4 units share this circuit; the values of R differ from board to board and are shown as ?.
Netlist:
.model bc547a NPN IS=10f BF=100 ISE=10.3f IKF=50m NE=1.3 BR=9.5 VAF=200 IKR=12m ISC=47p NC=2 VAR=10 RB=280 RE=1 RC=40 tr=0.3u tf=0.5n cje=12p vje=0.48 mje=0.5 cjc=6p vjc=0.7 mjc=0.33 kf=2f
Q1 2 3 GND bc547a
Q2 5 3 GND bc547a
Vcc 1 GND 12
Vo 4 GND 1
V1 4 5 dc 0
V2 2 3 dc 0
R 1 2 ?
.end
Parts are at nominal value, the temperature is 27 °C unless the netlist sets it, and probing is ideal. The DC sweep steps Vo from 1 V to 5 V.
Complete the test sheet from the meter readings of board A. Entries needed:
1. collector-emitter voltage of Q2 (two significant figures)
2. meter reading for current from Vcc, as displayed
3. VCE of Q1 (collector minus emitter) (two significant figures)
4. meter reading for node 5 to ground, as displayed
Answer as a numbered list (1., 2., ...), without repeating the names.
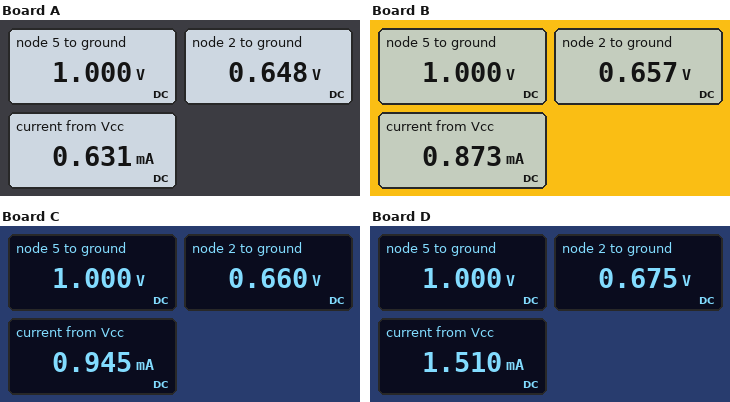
1. 1.0 V
2. 0.631 mA
3. 650 mV
4. 1.000 V
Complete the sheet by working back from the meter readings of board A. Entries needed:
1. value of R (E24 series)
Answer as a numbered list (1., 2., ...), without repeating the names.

1. 18 kΩ
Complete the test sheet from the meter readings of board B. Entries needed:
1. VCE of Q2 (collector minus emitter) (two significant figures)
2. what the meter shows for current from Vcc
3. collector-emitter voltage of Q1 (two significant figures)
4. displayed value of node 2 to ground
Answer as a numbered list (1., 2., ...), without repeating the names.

1. 1.0 V
2. 0.873 mA
3. 660 mV
4. 0.657 V
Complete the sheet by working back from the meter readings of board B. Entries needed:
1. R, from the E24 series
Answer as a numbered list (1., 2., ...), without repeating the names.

1. 13 kΩ
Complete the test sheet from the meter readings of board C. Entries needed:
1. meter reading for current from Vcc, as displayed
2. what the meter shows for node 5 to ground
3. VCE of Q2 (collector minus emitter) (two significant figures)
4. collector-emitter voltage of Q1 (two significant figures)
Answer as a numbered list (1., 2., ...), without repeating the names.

1. 0.945 mA
2. 1.000 V
3. 1.0 V
4. 660 mV
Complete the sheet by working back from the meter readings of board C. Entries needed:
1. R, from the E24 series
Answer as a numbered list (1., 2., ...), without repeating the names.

1. 12 kΩ
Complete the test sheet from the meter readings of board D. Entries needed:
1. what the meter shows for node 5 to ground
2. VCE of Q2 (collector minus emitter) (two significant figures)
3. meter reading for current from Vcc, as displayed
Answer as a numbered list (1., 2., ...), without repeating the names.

1. 1.000 V
2. 1.0 V
3. 1.510 mA
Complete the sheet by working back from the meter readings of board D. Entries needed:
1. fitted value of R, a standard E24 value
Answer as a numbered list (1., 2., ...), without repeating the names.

1. 7.5 kΩ
